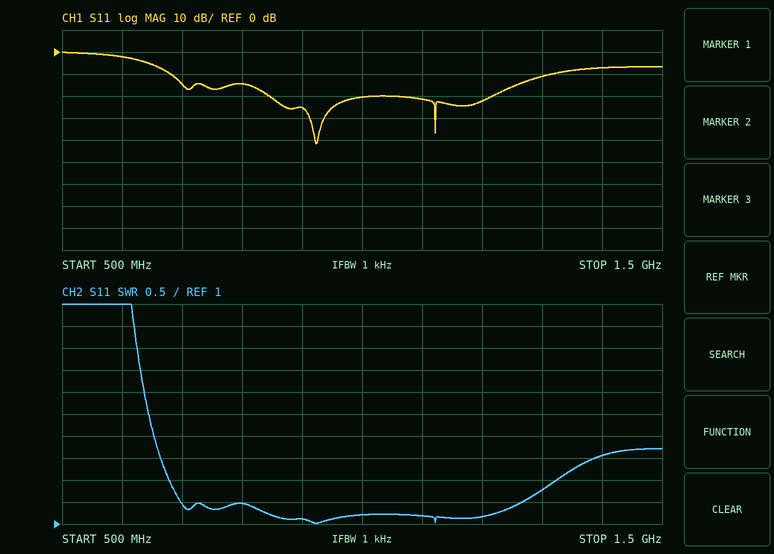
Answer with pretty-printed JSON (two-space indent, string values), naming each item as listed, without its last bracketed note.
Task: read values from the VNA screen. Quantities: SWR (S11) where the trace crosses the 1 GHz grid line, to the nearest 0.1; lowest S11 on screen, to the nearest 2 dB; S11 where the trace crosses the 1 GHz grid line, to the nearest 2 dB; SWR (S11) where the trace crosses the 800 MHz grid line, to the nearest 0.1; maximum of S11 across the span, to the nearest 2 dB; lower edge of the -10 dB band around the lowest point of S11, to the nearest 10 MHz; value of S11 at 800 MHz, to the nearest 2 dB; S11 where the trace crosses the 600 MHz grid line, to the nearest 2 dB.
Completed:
{
  "SWR (S11) where the trace crosses the 1 GHz grid line, to the nearest 0.1": "1.2",
  "lowest S11 on screen, to the nearest 2 dB": "-42 dB",
  "S11 where the trace crosses the 1 GHz grid line, to the nearest 2 dB": "-20 dB",
  "SWR (S11) where the trace crosses the 800 MHz grid line, to the nearest 0.1": "1.5",
  "maximum of S11 across the span, to the nearest 2 dB": "0 dB",
  "lower edge of the -10 dB band around the lowest point of S11, to the nearest 10 MHz": "680 MHz",
  "value of S11 at 800 MHz, to the nearest 2 dB": "-14 dB",
  "S11 where the trace crosses the 600 MHz grid line, to the nearest 2 dB": "-2 dB"
}
